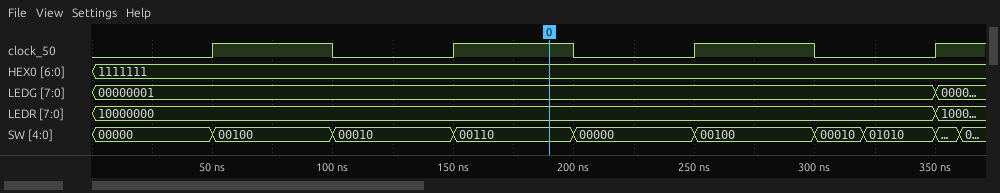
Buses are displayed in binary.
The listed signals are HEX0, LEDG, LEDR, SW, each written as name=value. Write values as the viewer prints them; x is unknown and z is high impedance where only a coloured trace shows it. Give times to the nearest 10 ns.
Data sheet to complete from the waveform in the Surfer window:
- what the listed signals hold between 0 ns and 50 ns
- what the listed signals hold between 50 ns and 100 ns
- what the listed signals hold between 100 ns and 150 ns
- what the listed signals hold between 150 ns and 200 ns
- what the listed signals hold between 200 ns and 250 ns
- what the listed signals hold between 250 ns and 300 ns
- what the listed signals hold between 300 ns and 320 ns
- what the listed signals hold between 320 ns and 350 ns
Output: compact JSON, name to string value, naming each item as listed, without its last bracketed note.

{"what the listed signals hold between 0 ns and 50 ns": "HEX0=1111111, LEDG=00000001, LEDR=10000000, SW=00000", "what the listed signals hold between 50 ns and 100 ns": "HEX0=1111111, LEDG=00000001, LEDR=10000000, SW=00100", "what the listed signals hold between 100 ns and 150 ns": "HEX0=1111111, LEDG=00000001, LEDR=10000000, SW=00010", "what the listed signals hold between 150 ns and 200 ns": "HEX0=1111111, LEDG=00000001, LEDR=10000000, SW=00110", "what the listed signals hold between 200 ns and 250 ns": "HEX0=1111111, LEDG=00000001, LEDR=10000000, SW=00000", "what the listed signals hold between 250 ns and 300 ns": "HEX0=1111111, LEDG=00000001, LEDR=10000000, SW=00100", "what the listed signals hold between 300 ns and 320 ns": "HEX0=1111111, LEDG=00000001, LEDR=10000000, SW=00010", "what the listed signals hold between 320 ns and 350 ns": "HEX0=1111111, LEDG=00000001, LEDR=10000000, SW=01010"}
